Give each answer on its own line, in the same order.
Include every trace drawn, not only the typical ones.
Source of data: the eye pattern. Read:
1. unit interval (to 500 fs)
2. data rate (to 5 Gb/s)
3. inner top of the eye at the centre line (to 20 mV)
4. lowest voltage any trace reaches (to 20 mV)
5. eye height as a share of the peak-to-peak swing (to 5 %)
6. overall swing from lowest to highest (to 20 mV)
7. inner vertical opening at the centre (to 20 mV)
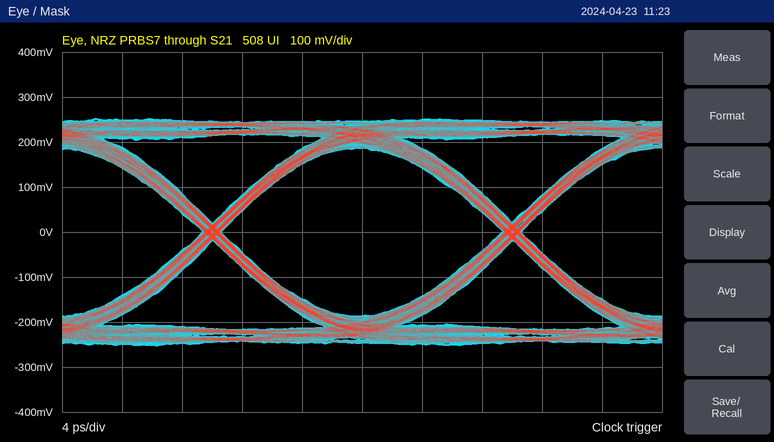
20.0 ps
50 Gb/s
180 mV
-260 mV
75 %
500 mV
380 mV
